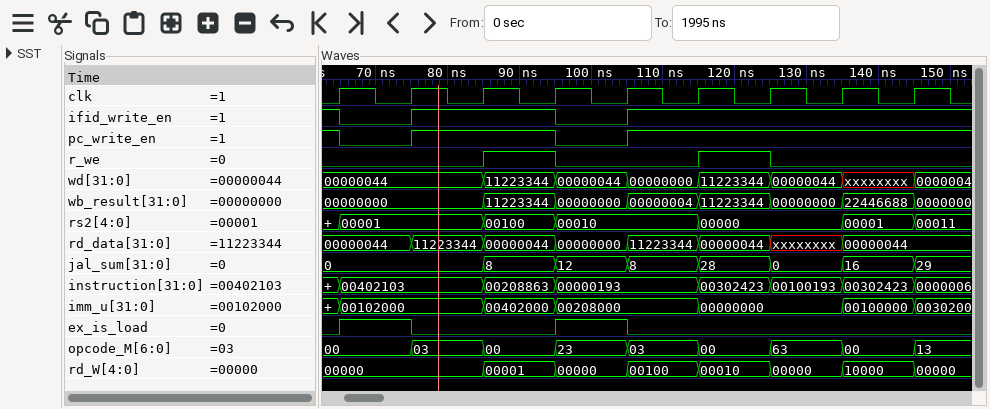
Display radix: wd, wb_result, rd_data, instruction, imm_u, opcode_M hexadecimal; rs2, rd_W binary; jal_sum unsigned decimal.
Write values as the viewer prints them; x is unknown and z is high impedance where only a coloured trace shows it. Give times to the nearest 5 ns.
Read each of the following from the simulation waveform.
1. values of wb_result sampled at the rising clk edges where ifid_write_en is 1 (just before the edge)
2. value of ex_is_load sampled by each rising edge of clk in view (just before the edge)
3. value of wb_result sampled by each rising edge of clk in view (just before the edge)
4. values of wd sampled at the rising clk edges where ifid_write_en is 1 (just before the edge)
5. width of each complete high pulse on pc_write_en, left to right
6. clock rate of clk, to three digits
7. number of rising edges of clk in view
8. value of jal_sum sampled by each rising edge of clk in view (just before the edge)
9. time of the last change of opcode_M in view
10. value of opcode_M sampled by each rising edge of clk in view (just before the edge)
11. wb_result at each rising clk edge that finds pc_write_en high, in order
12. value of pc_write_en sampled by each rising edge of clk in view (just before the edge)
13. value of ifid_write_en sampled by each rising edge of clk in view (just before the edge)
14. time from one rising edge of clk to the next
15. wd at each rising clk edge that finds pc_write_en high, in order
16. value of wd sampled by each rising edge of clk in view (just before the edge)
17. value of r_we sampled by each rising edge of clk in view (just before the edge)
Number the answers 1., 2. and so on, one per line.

1. 00000000, 00000000, 11223344, 00000004, 11223344, 00000000, 22446688
2. 0 1 0 0 1 0 0 0 0
3. 00000000, 00000000, 00000000, 11223344, 00000000, 00000004, 11223344, 00000000, 22446688
4. 00000044, 00000044, 11223344, 00000000, 11223344, 00000044, xxxxxxxx
5. 20 ns
6. 100 MHz
7. 9
8. 0, 0, 0, 8, 12, 8, 28, 0, 16
9. 145 ns
10. 00, 00, 03, 00, 23, 03, 00, 63, 00
11. 00000000, 00000000, 11223344, 00000004, 11223344, 00000000, 22446688
12. 1 0 1 1 0 1 1 1 1
13. 1 0 1 1 0 1 1 1 1
14. 10 ns
15. 00000044, 00000044, 11223344, 00000000, 11223344, 00000044, xxxxxxxx
16. 00000044, 00000044, 00000044, 11223344, 00000044, 00000000, 11223344, 00000044, xxxxxxxx
17. 0 0 0 1 0 0 1 0 0
